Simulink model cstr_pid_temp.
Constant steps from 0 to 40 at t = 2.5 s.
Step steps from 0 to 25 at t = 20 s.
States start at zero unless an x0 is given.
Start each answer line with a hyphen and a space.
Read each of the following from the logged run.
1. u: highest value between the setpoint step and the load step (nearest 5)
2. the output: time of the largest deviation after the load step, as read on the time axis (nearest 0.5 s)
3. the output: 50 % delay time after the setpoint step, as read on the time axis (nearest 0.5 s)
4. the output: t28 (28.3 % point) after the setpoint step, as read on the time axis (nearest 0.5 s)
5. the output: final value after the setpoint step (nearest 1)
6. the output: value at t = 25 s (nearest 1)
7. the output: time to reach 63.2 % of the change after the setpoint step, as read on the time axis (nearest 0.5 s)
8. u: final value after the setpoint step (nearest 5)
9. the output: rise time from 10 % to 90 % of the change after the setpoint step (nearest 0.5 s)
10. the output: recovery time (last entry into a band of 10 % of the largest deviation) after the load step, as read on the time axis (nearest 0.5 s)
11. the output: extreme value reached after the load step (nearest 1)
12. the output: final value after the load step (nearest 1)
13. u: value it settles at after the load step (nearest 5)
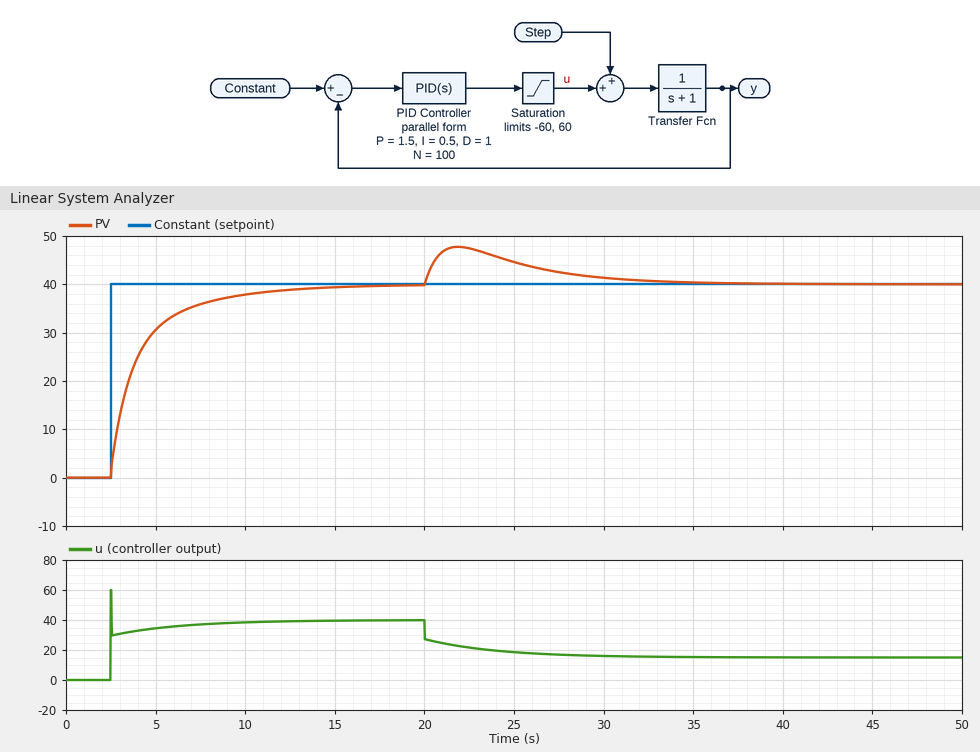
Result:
- 60
- 22.0 s
- 3.5 s
- 3.0 s
- 40
- 45
- 4.0 s
- 40
- 5.0 s
- 32.0 s
- 48
- 40
- 15
